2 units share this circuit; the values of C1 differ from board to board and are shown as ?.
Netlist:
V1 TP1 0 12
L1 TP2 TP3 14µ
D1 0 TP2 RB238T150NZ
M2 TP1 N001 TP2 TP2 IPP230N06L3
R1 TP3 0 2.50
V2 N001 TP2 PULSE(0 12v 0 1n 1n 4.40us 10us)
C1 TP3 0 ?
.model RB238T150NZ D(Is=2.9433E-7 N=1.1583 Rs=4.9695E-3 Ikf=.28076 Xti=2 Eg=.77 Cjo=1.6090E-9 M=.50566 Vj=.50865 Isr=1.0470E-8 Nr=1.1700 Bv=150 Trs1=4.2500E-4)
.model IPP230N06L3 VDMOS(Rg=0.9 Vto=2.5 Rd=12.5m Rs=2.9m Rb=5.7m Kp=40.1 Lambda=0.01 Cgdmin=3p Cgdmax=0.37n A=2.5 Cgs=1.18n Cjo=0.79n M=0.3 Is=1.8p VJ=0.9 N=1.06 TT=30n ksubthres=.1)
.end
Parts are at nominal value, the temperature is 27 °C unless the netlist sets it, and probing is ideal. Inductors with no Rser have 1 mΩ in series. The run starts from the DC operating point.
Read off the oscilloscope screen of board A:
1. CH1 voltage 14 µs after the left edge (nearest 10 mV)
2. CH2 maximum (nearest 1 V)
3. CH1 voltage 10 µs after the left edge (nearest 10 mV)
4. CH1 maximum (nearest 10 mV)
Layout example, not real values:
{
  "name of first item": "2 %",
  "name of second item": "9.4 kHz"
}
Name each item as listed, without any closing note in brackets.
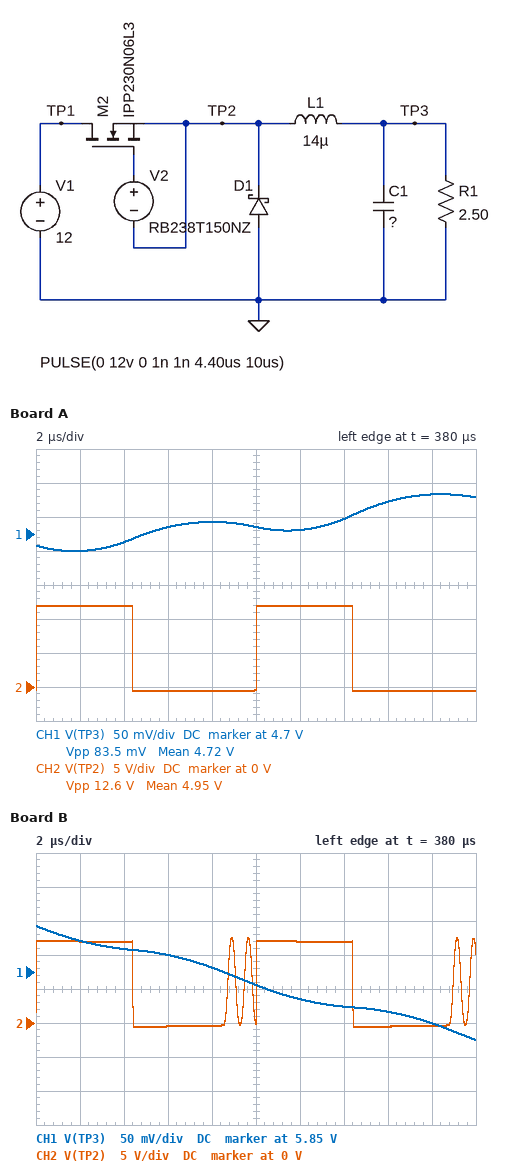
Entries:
{
  "CH1 voltage 14 µs after the left edge": "4.72 V",
  "CH2 maximum": "12 V",
  "CH1 voltage 10 µs after the left edge": "4.71 V",
  "CH1 maximum": "4.76 V"
}
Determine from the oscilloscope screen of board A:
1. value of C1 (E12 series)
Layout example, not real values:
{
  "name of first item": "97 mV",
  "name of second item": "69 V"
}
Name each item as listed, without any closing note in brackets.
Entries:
{
  "value of C1": "100 µF"
}
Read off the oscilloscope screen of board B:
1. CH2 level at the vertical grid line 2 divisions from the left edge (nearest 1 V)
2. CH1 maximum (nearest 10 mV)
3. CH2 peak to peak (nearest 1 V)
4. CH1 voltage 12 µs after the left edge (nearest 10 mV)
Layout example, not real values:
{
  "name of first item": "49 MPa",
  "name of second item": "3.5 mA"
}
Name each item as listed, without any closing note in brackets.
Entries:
{
  "CH2 level at the vertical grid line 2 divisions from the left edge": "12 V",
  "CH1 maximum": "5.92 V",
  "CH2 peak to peak": "13 V",
  "CH1 voltage 12 µs after the left edge": "5.81 V"
}
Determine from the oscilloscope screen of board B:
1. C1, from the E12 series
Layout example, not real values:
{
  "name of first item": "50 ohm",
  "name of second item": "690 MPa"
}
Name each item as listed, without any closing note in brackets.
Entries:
{
  "C1, from the E12 series": "180 µF"
}
